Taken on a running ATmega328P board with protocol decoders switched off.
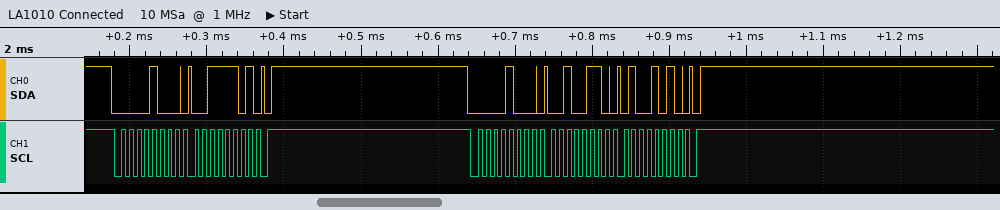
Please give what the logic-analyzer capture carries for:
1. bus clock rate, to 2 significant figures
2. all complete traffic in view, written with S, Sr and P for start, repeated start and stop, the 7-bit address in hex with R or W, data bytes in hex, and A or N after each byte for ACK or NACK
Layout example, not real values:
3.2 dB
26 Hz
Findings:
100 kHz
S 04W A 3D A P S 04W A 26 A 4A A P
